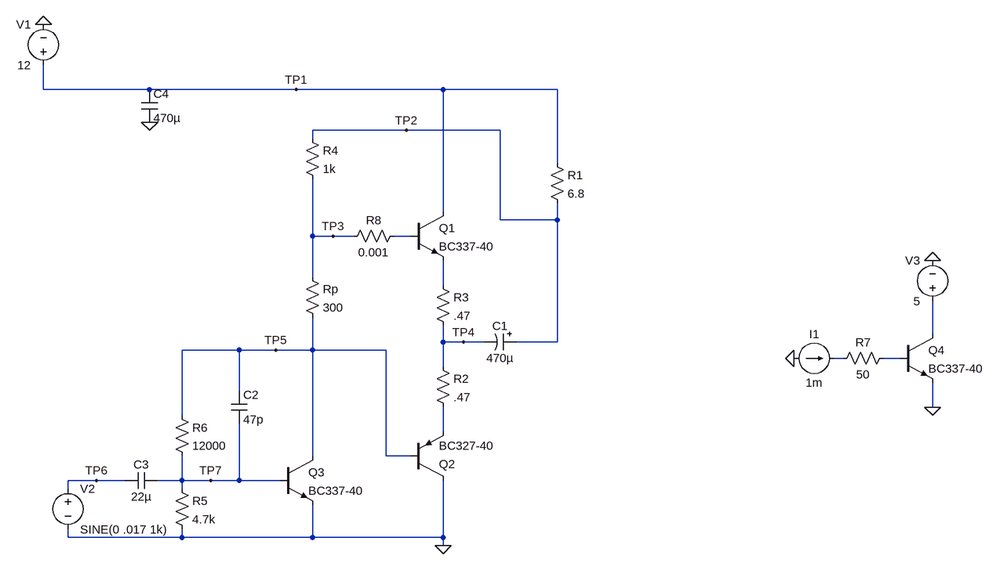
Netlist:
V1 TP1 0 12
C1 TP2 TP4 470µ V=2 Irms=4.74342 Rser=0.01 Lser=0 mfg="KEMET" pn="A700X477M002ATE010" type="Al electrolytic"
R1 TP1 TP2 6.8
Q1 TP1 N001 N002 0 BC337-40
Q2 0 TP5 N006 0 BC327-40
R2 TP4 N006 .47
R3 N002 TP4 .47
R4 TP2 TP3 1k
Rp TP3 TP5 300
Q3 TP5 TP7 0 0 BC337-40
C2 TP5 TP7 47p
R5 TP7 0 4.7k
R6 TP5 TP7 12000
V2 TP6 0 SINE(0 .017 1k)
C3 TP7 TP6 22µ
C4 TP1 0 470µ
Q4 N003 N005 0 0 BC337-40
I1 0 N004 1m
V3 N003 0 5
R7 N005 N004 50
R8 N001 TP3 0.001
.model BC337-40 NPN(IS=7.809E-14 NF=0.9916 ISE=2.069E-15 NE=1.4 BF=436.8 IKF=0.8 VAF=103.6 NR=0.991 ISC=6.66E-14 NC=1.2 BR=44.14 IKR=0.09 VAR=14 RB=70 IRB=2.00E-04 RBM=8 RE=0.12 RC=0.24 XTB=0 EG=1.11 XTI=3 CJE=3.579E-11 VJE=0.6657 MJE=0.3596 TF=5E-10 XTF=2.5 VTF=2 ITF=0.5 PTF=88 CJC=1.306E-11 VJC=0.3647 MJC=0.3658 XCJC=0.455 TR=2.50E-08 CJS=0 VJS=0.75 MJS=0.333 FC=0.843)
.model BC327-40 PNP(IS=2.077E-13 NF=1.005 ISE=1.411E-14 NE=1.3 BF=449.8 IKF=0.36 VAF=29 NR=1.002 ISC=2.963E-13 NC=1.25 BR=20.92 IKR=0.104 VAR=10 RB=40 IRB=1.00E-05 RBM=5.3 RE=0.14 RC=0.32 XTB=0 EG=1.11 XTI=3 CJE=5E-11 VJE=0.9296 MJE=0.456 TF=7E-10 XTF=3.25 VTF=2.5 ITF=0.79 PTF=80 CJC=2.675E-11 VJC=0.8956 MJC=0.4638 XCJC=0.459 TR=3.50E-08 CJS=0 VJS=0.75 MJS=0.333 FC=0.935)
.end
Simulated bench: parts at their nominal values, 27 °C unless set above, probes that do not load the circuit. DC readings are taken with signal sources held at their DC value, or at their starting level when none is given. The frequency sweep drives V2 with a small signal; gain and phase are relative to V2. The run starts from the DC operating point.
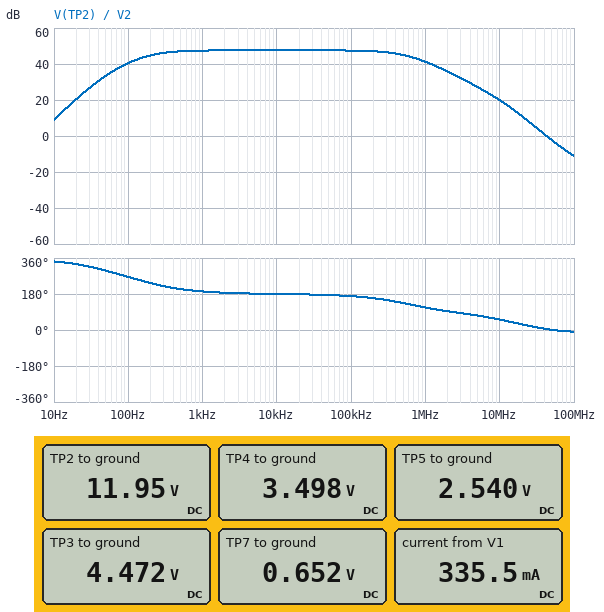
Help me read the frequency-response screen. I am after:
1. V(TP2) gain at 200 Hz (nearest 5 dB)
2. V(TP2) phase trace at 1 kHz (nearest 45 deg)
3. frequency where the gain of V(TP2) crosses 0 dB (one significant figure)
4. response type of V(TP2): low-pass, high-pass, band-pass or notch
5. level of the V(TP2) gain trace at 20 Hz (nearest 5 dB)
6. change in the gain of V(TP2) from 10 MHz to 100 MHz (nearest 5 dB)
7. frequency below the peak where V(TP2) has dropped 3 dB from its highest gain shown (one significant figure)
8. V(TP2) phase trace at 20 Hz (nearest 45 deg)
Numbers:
45 dB
180 deg
40 MHz
band-pass
20 dB
-30 dB
200 Hz
315 deg
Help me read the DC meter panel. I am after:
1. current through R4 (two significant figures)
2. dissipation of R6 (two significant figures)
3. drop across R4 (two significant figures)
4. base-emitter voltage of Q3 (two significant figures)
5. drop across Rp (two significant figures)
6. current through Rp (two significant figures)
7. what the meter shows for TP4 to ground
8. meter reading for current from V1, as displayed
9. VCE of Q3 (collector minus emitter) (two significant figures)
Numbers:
7.5 mA
300 µW
7.5 V
650 mV
1.9 V
6.4 mA
3.498 V
335.5 mA
2.5 V
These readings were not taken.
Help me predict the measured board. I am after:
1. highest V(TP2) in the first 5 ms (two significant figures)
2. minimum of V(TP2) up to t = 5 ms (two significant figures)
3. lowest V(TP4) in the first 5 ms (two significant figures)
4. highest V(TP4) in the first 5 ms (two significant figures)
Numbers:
16 V
9.4 V
1.2 V
7.5 V
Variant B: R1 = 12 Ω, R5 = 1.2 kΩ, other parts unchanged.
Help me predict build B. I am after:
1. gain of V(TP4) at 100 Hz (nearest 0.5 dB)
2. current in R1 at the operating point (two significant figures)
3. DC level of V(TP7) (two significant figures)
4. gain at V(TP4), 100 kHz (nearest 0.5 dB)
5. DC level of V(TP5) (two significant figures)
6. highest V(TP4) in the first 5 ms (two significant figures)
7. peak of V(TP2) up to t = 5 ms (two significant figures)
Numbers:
31.5 dB
3.8 mA
630 mV
35.0 dB
7.0 V
11 V
15 V
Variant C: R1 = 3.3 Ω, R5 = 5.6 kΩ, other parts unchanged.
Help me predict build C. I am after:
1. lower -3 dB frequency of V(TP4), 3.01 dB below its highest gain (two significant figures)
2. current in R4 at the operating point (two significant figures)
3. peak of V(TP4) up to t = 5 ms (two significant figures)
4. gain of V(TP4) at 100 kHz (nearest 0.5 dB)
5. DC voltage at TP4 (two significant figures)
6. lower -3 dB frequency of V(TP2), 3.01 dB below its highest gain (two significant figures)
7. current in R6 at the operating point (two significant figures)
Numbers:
70 Hz
7.7 mA
5.4 V
42.0 dB
3.3 V
120 Hz
140 µA
